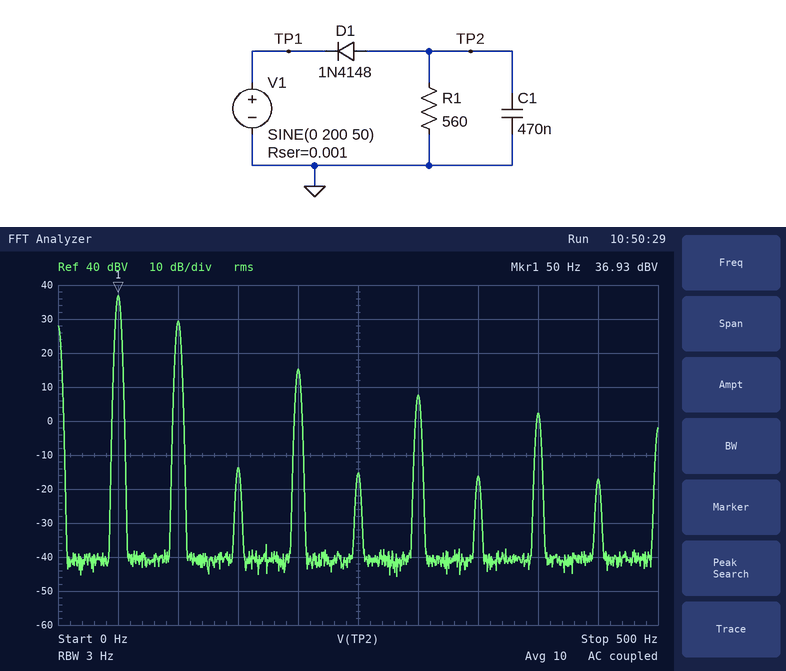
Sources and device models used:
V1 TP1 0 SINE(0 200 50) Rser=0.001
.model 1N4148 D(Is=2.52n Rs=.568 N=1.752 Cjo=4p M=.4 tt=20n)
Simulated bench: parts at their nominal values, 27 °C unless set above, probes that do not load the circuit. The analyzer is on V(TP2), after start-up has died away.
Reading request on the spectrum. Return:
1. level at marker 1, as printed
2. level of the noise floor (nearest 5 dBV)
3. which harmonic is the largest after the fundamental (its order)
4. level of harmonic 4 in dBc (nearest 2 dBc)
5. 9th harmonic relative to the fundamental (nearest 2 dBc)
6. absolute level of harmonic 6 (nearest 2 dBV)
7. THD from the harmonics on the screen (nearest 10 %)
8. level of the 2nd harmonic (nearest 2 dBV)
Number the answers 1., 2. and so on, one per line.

1. 36.93 dBV
2. -40 dBV
3. 2
4. -22 dBc
5. -54 dBc
6. 8 dBV
7. 40 %
8. 30 dBV
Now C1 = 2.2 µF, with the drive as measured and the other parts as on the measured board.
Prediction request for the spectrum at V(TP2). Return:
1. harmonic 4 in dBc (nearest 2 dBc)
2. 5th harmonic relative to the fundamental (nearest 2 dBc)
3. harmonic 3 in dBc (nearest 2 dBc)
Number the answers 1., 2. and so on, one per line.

1. -24 dBc
2. -34 dBc
3. -30 dBc
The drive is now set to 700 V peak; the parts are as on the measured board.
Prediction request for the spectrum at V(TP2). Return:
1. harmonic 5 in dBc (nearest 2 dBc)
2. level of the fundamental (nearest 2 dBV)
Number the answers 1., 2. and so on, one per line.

1. -54 dBc
2. 48 dBV
